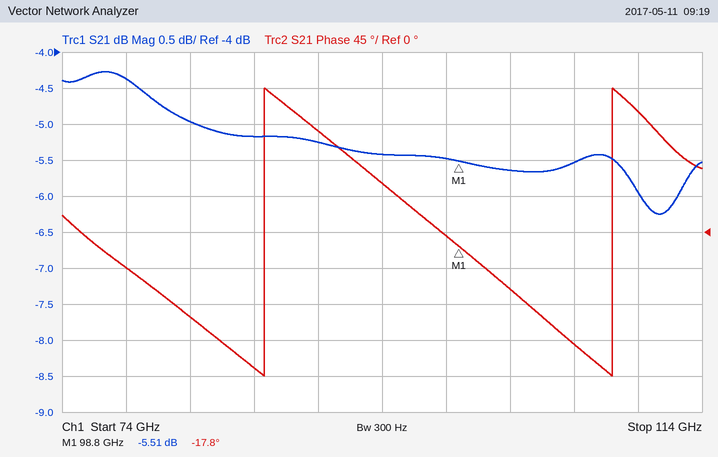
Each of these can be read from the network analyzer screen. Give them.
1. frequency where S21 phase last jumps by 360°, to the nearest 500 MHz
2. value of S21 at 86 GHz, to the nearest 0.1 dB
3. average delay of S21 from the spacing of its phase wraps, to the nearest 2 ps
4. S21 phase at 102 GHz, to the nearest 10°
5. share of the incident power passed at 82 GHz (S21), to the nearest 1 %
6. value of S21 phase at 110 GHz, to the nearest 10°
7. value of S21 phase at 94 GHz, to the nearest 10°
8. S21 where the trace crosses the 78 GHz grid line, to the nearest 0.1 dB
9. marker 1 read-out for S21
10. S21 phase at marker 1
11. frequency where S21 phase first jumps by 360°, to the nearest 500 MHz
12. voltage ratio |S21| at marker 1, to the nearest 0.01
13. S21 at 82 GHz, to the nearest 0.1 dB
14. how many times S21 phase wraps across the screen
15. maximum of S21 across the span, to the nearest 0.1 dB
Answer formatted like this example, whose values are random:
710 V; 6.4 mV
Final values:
108.5 GHz; -5.2 dB; 46 ps; -70°; 32 %; 150°; 60°; -4.4 dB; -5.51 dB; -17.8°; 86.5 GHz; 0.53; -5.0 dB; 2; -4.3 dB
